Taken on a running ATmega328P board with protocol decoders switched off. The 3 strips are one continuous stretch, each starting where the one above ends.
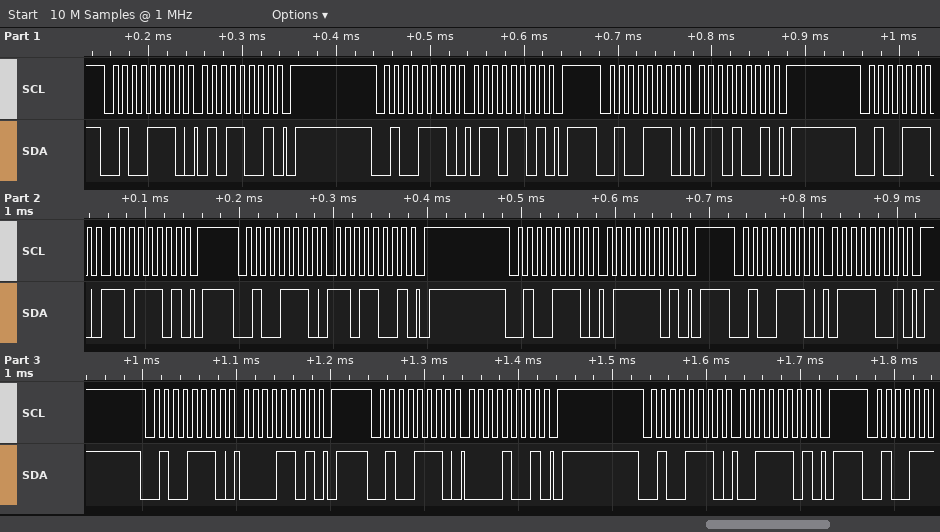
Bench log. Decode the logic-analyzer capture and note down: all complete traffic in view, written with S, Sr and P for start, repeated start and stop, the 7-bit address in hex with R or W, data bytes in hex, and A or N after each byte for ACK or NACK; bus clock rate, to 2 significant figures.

S 27W A 59 A P S 27W A 6D A P S 27W A 69 A P S 27W A DD A P S 27W A D9 A P S 27W A 7D A P S 27W A 79 A P S 27W A 0D A P S 27W A 09 A P S 27W A 3D A P
100 kHz
